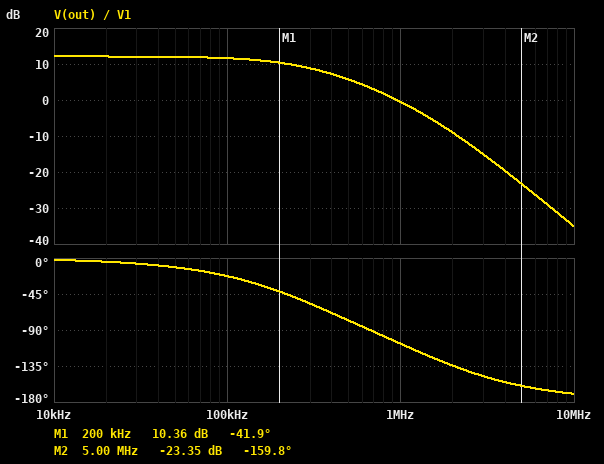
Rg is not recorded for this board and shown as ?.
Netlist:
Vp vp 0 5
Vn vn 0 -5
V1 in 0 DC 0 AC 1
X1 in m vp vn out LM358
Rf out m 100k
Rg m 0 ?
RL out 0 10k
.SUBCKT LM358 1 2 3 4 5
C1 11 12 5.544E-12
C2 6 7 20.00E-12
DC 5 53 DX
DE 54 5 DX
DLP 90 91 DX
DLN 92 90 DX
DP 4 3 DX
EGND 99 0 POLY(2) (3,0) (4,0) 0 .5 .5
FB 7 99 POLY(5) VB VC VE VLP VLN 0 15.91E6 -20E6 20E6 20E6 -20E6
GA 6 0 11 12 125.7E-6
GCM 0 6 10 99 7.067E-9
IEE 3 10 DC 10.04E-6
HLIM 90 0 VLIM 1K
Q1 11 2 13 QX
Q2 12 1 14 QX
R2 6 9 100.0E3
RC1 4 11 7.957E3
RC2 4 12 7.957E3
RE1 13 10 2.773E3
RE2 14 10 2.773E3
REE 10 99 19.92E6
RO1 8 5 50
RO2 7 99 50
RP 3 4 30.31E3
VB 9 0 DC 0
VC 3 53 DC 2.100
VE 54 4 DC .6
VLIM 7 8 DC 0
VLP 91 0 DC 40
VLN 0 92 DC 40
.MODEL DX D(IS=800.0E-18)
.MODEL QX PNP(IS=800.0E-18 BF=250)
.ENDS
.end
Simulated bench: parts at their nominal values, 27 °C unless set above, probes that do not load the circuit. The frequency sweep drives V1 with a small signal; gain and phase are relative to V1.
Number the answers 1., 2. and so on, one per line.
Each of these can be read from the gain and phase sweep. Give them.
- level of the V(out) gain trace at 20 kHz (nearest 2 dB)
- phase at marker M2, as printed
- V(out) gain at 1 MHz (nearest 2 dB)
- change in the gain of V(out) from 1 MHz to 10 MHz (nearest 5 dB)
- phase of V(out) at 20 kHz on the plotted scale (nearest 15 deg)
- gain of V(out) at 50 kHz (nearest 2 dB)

1. 12 dB
2. -159.8 deg
3. 0 dB
4. -35 dB
5. 0 deg
6. 12 dB
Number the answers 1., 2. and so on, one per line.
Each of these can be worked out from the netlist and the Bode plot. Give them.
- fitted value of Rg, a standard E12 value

1. 33 kΩ
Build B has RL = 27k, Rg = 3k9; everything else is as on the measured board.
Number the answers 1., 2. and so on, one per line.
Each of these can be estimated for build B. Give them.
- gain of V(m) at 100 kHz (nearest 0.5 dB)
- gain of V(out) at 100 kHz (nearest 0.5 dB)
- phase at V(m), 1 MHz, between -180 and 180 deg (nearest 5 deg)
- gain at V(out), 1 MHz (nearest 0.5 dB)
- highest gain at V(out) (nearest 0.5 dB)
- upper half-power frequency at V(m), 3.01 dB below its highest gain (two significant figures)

1. -9.0 dB
2. 19.5 dB
3. -115 deg
4. -1.0 dB
5. 28.5 dB
6. 38 kHz
